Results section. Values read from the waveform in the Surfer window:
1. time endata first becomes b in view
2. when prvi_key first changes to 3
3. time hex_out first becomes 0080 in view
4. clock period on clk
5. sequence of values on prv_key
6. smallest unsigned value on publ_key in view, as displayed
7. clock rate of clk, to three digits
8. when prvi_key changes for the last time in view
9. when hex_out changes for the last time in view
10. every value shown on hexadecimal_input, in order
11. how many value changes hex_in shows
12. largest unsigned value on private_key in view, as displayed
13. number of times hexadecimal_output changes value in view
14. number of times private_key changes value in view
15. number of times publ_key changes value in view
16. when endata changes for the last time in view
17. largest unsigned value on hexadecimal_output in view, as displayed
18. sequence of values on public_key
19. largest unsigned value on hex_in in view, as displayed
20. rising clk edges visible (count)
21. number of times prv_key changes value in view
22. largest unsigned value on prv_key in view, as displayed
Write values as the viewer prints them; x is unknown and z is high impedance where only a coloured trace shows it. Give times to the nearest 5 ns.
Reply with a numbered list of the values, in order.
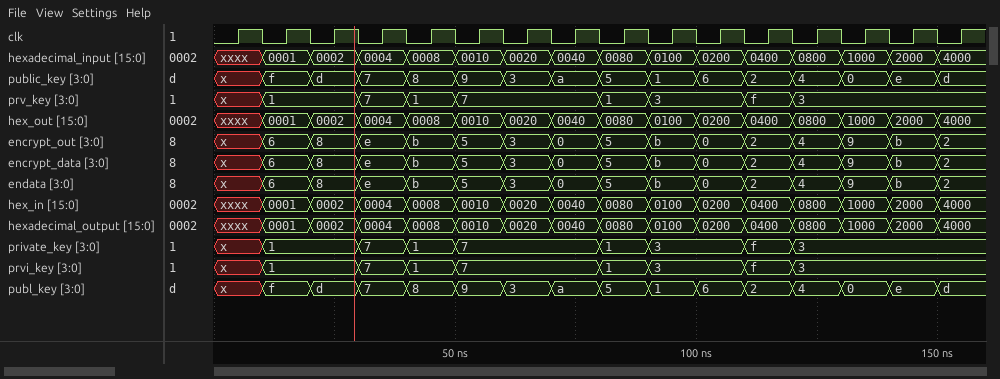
1. 40 ns
2. 90 ns
3. 80 ns
4. 10 ns
5. x, 1, 7, 1, 7, 1, 3, f, 3
6. 0
7. 100 MHz
8. 120 ns
9. 150 ns
10. xxxx, 0001, 0002, 0004, 0008, 0010, 0020, 0040, 0080, 0100, 0200, 0400, 0800, 1000, 2000, 4000
11. 15
12. f
13. 15
14. 8
15. 15
16. 150 ns
17. 4000
18. x, f, d, 7, 8, 9, 3, a, 5, 1, 6, 2, 4, 0, e, d
19. 4000
20. 16
21. 8
22. f
